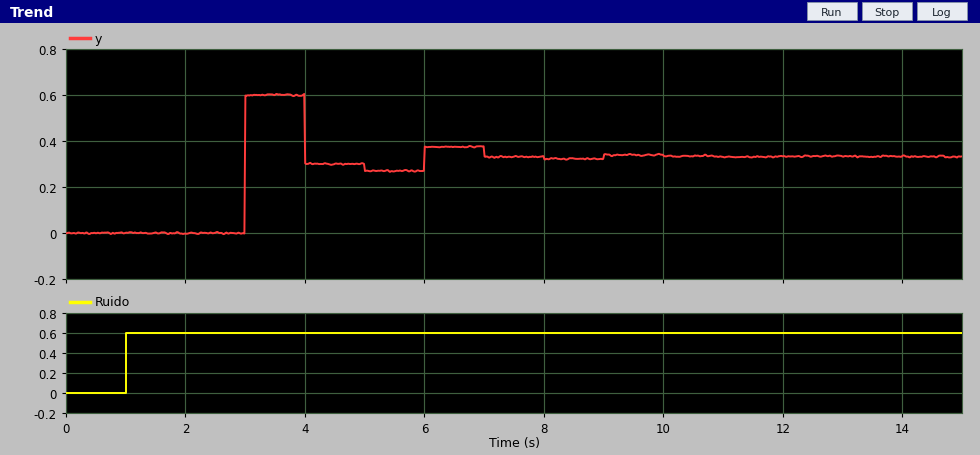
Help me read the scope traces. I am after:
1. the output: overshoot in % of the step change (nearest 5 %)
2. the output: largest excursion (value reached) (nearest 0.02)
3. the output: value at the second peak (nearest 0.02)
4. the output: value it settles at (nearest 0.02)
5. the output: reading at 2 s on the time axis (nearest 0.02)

80 %
0.60
0.38
0.34
0.00
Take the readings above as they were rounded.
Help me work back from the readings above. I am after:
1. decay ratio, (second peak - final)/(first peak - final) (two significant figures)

0.15
